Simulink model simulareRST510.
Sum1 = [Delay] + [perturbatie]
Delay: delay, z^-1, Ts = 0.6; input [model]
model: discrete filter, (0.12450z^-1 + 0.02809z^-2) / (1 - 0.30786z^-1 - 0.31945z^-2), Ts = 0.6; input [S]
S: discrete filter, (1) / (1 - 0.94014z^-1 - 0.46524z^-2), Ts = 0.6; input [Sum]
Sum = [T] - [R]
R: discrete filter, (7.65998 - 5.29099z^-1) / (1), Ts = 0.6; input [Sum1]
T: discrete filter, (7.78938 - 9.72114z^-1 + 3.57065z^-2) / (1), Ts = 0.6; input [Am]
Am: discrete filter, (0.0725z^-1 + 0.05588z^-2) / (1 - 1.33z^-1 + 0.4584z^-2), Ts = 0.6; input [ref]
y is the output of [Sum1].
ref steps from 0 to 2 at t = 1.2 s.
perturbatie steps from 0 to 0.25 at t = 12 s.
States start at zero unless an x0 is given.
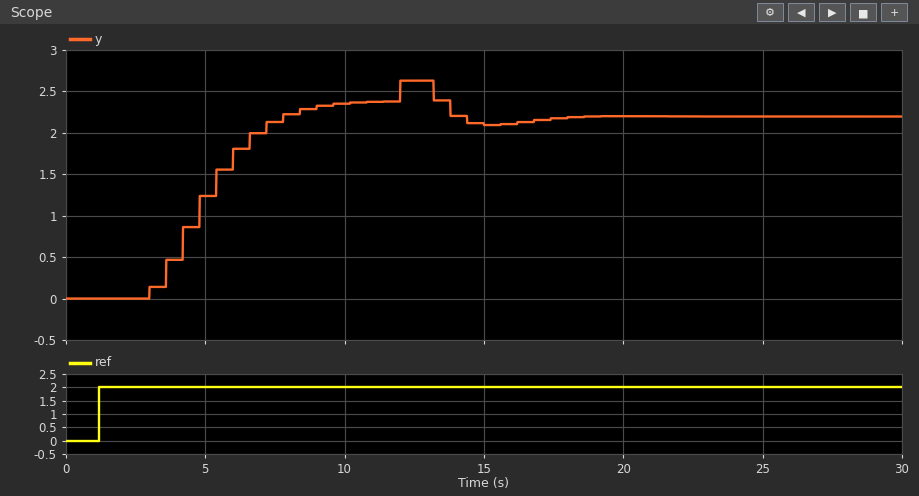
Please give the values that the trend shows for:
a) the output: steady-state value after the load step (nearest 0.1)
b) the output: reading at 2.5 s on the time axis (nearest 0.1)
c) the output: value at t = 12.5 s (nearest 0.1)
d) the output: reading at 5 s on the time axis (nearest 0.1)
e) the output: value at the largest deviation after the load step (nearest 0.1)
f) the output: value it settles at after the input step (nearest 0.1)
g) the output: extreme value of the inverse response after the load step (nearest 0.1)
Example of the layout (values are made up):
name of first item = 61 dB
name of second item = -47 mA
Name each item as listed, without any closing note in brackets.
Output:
the output: steady-state value after the load step = 2.2
the output: reading at 2.5 s on the time axis = 0.0
the output: value at t = 12.5 s = 2.6
the output: reading at 5 s on the time axis = 1.2
the output: value at the largest deviation after the load step = 2.1
the output: value it settles at after the input step = 2.4
the output: extreme value of the inverse response after the load step = 2.6
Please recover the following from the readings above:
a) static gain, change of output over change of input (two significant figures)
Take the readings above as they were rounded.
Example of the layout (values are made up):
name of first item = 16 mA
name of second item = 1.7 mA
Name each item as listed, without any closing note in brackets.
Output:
static gain, change of output over change of input = 1.2
